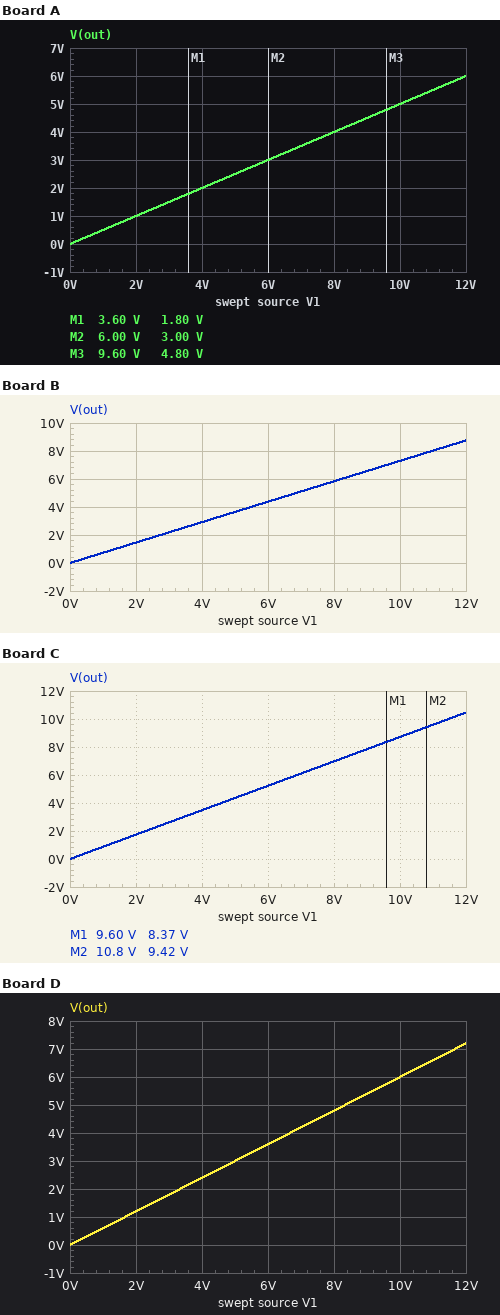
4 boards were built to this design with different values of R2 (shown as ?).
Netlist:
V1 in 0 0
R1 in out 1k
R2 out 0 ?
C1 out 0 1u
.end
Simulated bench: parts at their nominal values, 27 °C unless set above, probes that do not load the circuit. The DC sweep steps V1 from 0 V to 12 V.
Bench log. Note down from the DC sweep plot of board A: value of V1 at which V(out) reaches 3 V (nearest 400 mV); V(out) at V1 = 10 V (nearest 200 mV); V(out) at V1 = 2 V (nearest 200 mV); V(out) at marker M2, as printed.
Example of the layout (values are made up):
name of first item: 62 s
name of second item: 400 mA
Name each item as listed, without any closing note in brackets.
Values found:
value of V1 at which V(out) reaches 3 V: 6.0 V
V(out) at V1 = 10 V: 5.0 V
V(out) at V1 = 2 V: 1.0 V
V(out) at marker M2, as printed: 3.00 V
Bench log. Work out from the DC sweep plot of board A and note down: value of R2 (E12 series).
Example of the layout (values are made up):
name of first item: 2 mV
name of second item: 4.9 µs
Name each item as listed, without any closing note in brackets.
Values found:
value of R2: 1 kΩ
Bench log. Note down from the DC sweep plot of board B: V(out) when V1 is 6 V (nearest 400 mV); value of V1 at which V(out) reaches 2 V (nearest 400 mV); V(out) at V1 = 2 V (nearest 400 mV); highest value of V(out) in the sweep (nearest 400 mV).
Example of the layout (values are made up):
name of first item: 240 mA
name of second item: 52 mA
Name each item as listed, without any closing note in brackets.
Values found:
V(out) when V1 is 6 V: 4.4 V
value of V1 at which V(out) reaches 2 V: 2.8 V
V(out) at V1 = 2 V: 1.6 V
highest value of V(out) in the sweep: 8.8 V
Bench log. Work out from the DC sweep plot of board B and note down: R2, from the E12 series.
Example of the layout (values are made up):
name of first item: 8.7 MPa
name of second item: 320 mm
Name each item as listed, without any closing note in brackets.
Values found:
R2, from the E12 series: 2.7 kΩ
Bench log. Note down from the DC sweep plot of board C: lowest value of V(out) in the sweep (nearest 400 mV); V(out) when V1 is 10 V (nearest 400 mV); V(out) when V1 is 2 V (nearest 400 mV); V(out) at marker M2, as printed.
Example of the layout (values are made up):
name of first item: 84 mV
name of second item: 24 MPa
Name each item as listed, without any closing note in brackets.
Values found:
lowest value of V(out) in the sweep: 0 V
V(out) when V1 is 10 V: 8.8 V
V(out) when V1 is 2 V: 1.6 V
V(out) at marker M2, as printed: 9.42 V
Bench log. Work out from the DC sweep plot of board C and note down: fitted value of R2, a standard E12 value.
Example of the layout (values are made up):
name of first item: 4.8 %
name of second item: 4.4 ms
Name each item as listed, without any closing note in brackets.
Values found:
fitted value of R2, a standard E12 value: 6.8 kΩ
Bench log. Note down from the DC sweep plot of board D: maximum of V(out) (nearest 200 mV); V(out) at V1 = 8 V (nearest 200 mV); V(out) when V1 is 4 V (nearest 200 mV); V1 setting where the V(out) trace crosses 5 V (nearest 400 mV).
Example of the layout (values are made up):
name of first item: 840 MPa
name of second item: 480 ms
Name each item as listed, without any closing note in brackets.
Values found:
maximum of V(out): 7.2 V
V(out) at V1 = 8 V: 4.8 V
V(out) when V1 is 4 V: 2.4 V
V1 setting where the V(out) trace crosses 5 V: 8.4 V
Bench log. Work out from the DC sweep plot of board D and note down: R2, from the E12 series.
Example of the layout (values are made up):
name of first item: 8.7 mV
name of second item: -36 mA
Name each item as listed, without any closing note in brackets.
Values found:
R2, from the E12 series: 1.5 kΩ
